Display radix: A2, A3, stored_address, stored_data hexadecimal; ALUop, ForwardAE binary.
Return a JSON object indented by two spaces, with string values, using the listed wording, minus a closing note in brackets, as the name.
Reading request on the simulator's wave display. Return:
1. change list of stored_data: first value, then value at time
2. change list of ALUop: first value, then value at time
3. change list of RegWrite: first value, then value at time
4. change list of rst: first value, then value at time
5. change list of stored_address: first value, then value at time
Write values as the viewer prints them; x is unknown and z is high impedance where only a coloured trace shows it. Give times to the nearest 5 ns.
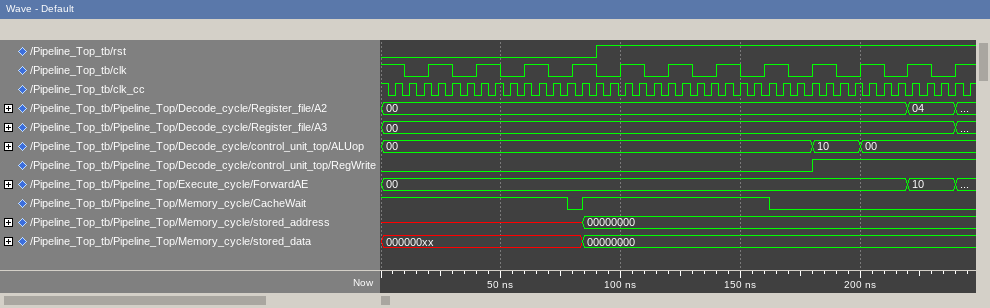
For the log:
{
  "change list of stored_data: first value, then value at time": "000000xx, 00000000 at 85 ns",
  "change list of ALUop: first value, then value at time": "00, 10 at 180 ns, 00 at 200 ns",
  "change list of RegWrite: first value, then value at time": "0, 1 at 180 ns",
  "change list of rst: first value, then value at time": "0, 1 at 90 ns",
  "change list of stored_address: first value, then value at time": "x, 00000000 at 85 ns"
}
